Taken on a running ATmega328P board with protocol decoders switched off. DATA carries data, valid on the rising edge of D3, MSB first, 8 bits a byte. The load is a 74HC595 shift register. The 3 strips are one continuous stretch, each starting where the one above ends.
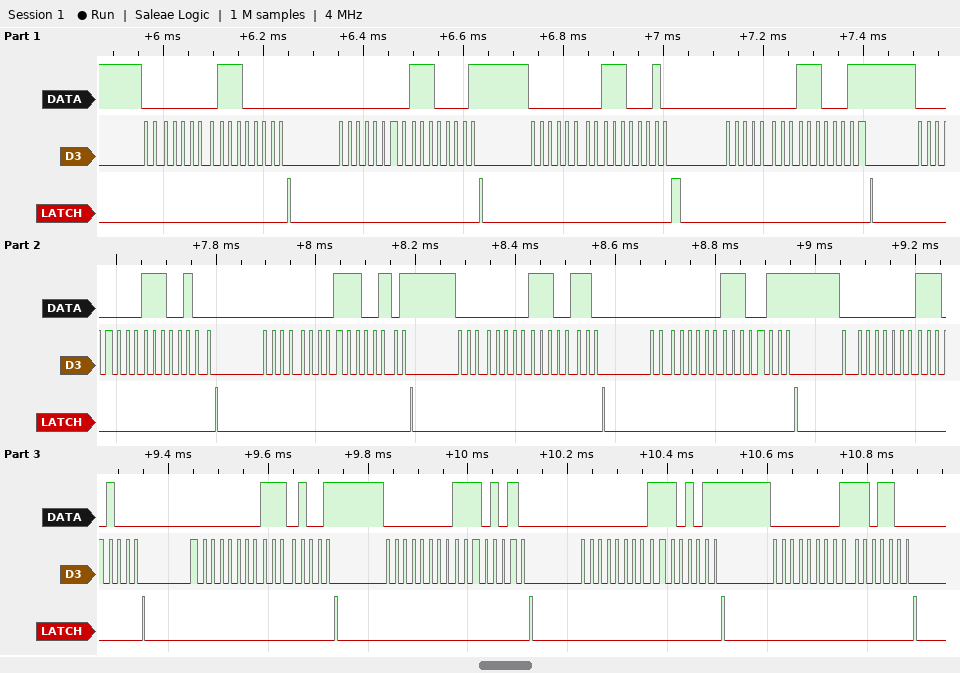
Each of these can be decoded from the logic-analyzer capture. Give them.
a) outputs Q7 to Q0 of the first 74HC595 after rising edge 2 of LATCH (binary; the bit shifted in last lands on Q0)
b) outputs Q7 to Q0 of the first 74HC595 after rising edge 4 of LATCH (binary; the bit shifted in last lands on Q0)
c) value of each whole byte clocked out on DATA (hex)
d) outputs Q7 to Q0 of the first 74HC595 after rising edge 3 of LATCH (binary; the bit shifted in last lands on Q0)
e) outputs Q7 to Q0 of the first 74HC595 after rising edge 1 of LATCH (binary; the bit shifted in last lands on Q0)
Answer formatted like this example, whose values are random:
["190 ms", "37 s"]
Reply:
["11100001", "11100011", "00 E0 00 E1 00 E2 00 E3 00 E4 00 E5 00 E6 00 E7 00 E8 00 E9 00 EA 00 EB 00 EC", "11100010", "11100000"]
